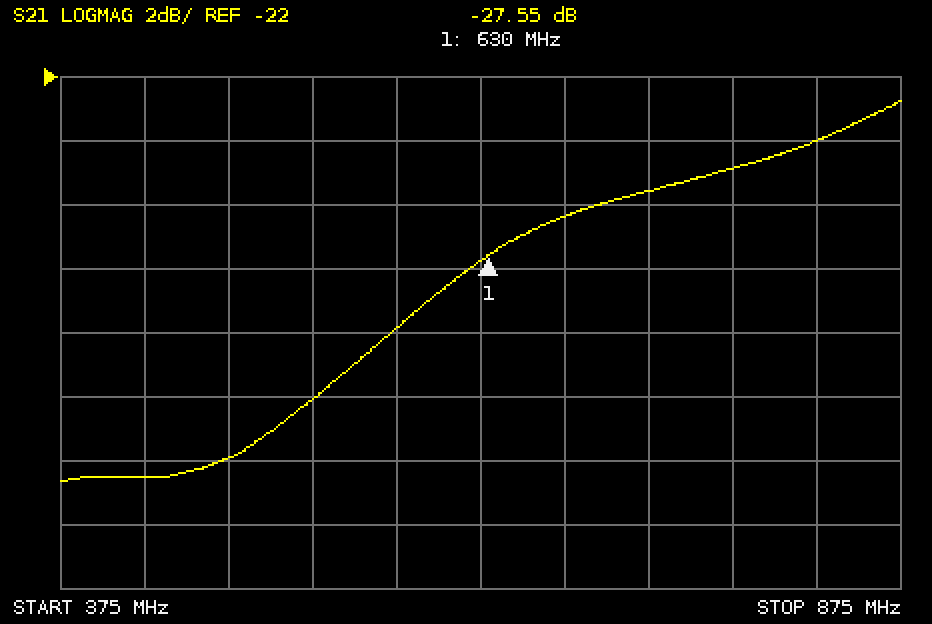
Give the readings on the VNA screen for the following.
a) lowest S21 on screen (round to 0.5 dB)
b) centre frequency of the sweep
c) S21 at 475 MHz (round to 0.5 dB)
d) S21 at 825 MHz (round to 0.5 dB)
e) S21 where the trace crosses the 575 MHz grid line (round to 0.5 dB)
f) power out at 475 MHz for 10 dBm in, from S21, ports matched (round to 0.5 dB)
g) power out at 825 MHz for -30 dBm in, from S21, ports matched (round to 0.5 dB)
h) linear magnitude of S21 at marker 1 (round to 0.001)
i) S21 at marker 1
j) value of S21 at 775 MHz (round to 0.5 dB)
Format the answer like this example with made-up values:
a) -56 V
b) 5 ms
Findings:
a) -34.5 dB
b) 625 MHz
c) -34.0 dB
d) -24.0 dB
e) -30.0 dB
f) -24.0 dBm
g) -54.0 dBm
h) 0.042
i) -27.55 dB
j) -25.0 dB
